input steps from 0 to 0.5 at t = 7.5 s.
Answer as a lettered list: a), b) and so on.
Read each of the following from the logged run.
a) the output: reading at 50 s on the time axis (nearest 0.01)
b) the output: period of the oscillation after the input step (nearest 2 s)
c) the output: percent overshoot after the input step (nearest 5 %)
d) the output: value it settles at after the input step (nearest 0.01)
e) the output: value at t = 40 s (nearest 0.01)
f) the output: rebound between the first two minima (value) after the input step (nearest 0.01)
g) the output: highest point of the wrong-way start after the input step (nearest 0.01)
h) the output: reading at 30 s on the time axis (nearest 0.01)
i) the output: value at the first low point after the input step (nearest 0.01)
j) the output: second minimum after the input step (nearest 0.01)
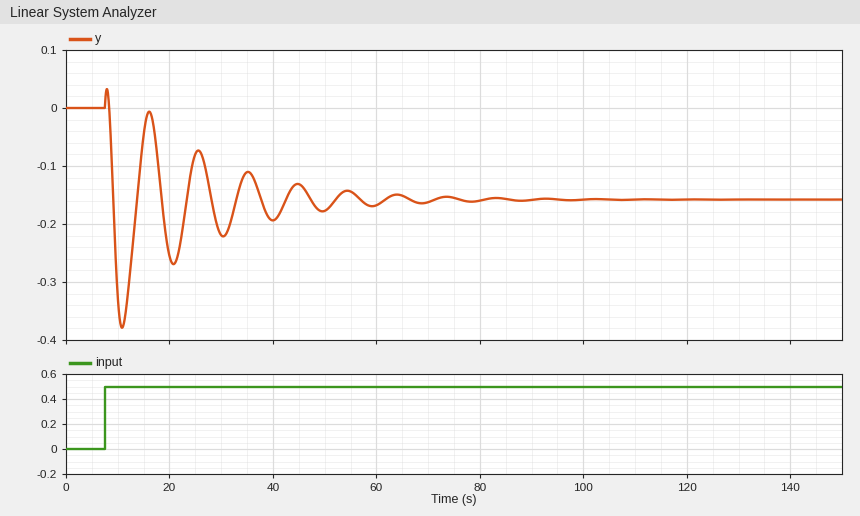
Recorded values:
a) -0.18
b) 10 s
c) 140 %
d) -0.16
e) -0.19
f) -0.01
g) 0.03
h) -0.22
i) -0.38
j) -0.27
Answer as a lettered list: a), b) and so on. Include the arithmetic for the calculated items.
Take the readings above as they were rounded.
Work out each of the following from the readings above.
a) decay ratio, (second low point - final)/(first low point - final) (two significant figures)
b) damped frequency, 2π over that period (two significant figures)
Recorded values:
a) (-0.27 - (-0.16)) / (-0.38 - (-0.16)) = 0.50
b) 2π / 10 = 0.63 rad/s
